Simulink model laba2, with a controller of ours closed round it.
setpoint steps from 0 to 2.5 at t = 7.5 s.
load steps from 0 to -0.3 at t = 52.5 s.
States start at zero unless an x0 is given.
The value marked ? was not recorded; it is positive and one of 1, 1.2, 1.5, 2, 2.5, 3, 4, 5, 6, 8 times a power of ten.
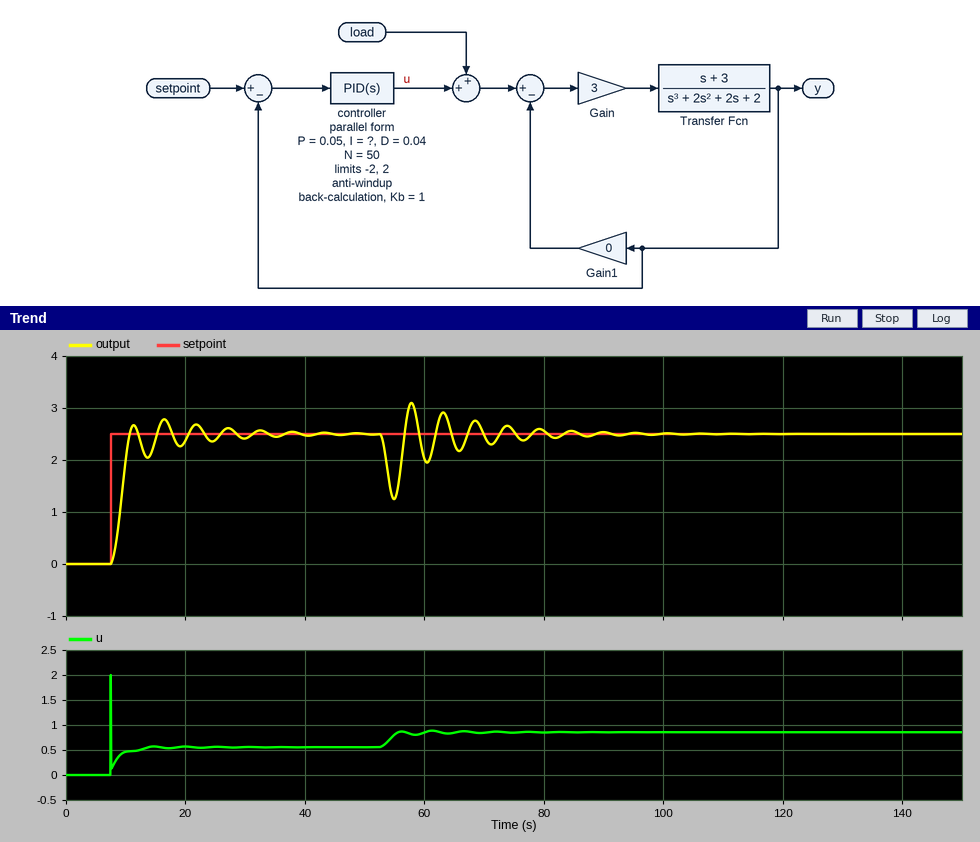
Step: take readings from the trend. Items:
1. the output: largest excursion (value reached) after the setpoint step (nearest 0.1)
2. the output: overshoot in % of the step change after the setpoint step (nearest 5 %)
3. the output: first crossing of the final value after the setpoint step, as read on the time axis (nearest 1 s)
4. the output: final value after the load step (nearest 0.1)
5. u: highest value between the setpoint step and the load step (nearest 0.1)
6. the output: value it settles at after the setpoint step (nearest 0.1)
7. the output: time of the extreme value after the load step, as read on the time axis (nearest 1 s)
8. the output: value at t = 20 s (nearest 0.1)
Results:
2.8
10 %
11 s
2.5
2.0
2.5
55 s
2.4
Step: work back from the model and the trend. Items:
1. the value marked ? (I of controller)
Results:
0.12
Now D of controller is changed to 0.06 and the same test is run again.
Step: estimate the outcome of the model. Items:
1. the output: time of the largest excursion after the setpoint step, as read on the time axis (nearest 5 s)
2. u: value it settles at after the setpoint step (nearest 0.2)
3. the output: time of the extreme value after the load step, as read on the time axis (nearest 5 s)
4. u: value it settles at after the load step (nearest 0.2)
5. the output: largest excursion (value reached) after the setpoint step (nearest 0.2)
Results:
15 s
0.6
55 s
0.8
2.6
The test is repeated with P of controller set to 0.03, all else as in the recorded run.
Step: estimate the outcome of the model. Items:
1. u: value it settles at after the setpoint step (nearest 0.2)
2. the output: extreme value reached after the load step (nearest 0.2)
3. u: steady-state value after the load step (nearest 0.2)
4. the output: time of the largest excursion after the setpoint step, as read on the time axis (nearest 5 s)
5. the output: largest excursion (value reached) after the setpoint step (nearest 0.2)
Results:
0.6
1.2
0.8
15 s
2.8
